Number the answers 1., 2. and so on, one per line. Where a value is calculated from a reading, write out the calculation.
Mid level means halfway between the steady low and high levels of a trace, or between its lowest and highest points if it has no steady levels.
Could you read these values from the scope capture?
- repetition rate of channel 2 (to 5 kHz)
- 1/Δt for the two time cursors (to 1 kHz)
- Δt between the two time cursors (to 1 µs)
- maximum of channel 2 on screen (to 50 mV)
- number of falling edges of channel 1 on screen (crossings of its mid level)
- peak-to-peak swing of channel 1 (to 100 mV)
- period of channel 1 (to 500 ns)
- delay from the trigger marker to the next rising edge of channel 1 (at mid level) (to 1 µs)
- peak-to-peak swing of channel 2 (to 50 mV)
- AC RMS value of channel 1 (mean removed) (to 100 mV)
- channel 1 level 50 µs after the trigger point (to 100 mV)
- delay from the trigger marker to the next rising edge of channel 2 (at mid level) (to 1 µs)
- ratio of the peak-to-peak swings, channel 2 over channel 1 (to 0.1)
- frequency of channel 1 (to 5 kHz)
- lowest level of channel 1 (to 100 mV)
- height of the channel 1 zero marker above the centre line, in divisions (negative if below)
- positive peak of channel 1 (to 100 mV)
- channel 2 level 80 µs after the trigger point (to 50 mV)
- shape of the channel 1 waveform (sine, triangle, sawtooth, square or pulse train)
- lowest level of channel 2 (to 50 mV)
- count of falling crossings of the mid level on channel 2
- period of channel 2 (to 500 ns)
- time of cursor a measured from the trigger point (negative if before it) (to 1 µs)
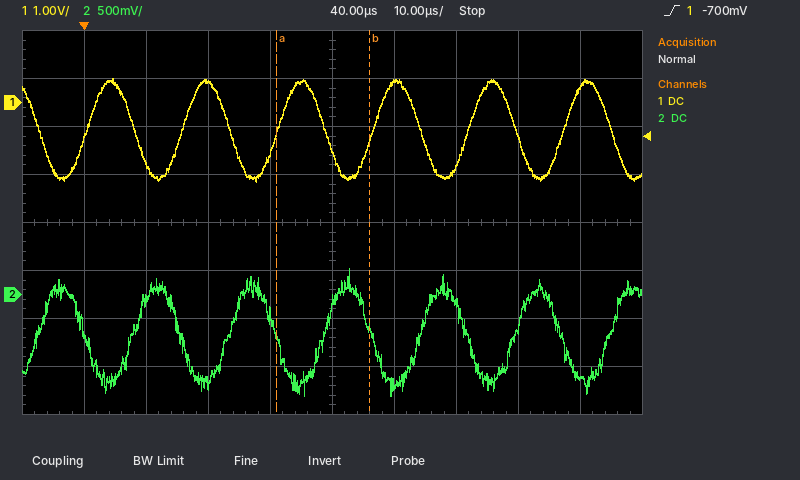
1. 1 / 15.5 µs ≈ 65 kHz
2. 1 / 15 µs ≈ 67 kHz
3. 15 µs
4. 250 mV
5. 7
6. 500 mV − (-1.6 V) = 2.1 V
7. 15.5 µs
8. 16 µs
9. 250 mV − (-1.05 V) = 1.30 V
10. 2.1 V / (2√2) ≈ 742 mV, so 700 mV to the nearest 100 mV
11. 400 mV
12. 8 µs
13. 1.30 V / 2.1 V ≈ 0.6
14. 1 / 15.5 µs ≈ 65 kHz
15. -1.6 V
16. +2.5 div
17. 500 mV
18. -850 mV
19. sine
20. -1.05 V
21. 6
22. 15.5 µs
23. +31 µs
